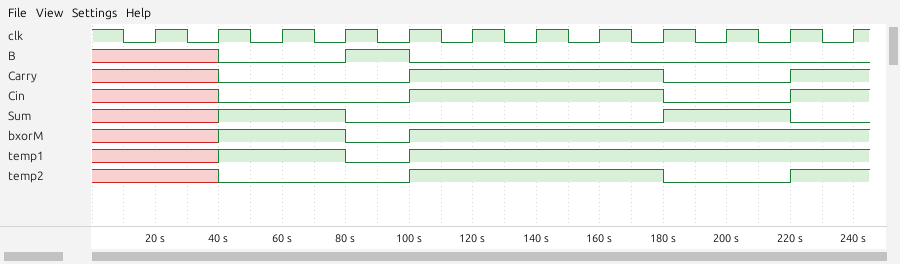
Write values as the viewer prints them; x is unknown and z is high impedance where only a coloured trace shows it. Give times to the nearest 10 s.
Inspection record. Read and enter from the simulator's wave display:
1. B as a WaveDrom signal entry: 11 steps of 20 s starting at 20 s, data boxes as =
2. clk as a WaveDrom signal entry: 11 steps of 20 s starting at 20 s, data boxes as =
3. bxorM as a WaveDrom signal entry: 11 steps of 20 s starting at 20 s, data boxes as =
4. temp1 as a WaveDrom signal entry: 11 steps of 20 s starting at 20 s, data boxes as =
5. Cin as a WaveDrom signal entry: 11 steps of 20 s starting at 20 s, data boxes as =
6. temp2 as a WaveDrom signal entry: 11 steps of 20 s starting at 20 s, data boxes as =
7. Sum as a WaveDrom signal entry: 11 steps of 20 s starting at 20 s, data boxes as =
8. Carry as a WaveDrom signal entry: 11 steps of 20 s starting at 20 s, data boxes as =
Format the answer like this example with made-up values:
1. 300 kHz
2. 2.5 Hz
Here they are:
1. {name: 'B', wave: 'x0.10......'}
2. {name: 'clk', wave: 'p..........'}
3. {name: 'bxorM', wave: 'x1.01......'}
4. {name: 'temp1', wave: 'x1.01......'}
5. {name: 'Cin', wave: 'x0..1...0.1'}
6. {name: 'temp2', wave: 'x0..1...0.1'}
7. {name: 'Sum', wave: 'x1.0....1.0'}
8. {name: 'Carry', wave: 'x0..1...0.1'}
